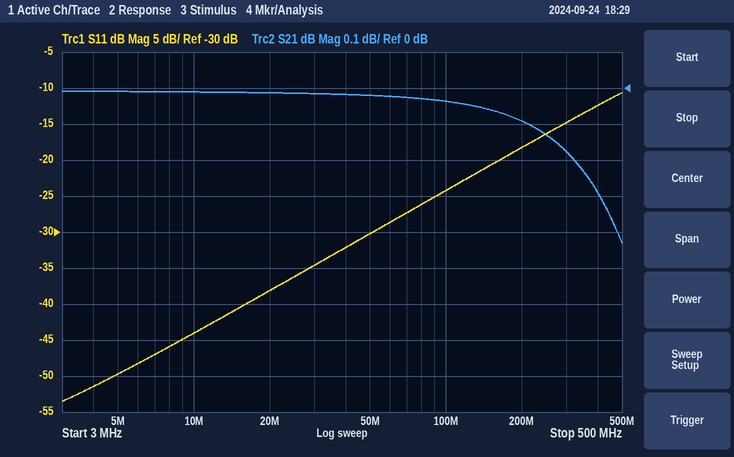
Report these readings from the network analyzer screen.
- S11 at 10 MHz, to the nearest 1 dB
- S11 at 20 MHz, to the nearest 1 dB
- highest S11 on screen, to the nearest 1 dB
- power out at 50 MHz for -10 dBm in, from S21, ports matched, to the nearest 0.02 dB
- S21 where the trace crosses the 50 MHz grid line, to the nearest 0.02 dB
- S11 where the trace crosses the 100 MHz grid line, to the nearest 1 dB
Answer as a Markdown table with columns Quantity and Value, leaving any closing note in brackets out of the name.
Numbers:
| Quantity | Value |
|---|---|
| S11 at 10 MHz, to the nearest 1 dB | -44 dB |
| S11 at 20 MHz, to the nearest 1 dB | -38 dB |
| highest S11 on screen, to the nearest 1 dB | -11 dB |
| power out at 50 MHz for -10 dBm in, from S21, ports matched, to the nearest 0.02 dB | -10.02 dBm |
| S21 where the trace crosses the 50 MHz grid line, to the nearest 0.02 dB | -0.02 dB |
| S11 where the trace crosses the 100 MHz grid line, to the nearest 1 dB | -24 dB |
